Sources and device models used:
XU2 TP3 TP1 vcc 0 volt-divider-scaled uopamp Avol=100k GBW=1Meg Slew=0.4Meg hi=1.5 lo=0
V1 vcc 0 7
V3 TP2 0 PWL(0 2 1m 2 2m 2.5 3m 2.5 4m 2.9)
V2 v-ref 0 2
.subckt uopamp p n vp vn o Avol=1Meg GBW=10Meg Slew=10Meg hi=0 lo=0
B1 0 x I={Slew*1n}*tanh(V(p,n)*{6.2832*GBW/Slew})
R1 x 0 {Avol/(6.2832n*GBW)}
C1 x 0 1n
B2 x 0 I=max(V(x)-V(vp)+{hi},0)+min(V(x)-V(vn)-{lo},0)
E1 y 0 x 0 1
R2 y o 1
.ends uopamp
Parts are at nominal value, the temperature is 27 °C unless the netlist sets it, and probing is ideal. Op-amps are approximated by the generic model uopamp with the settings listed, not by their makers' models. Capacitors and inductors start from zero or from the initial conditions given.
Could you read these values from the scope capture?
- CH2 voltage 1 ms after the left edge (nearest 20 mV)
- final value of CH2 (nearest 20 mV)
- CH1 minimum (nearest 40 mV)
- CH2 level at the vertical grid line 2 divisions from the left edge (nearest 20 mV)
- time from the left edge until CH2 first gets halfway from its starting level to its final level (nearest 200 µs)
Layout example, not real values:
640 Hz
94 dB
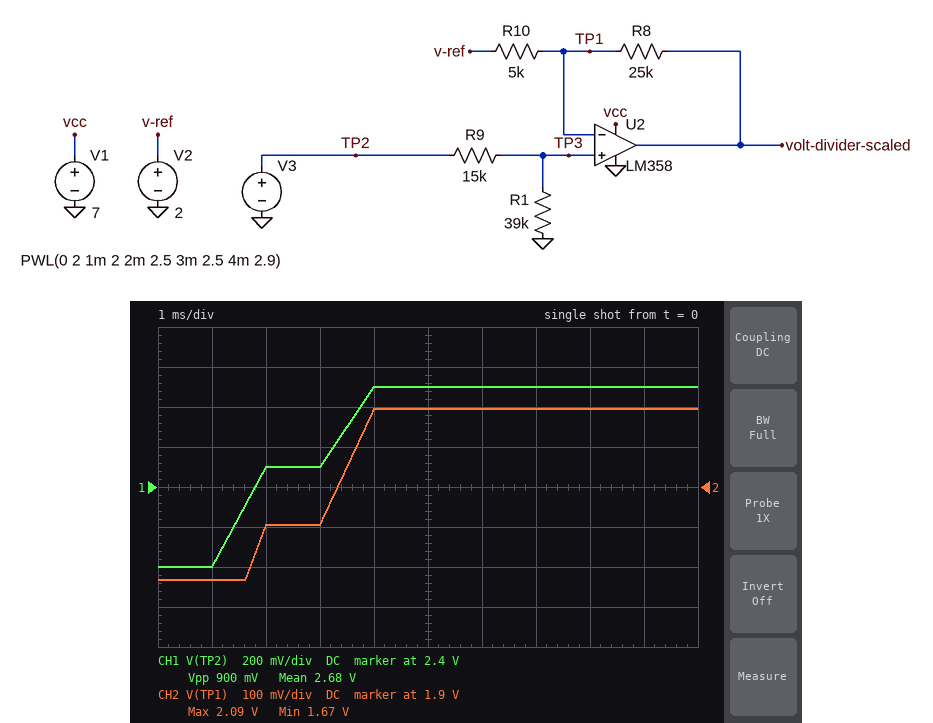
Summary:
1.66 V
2.10 V
2.00 V
1.80 V
3.2 ms
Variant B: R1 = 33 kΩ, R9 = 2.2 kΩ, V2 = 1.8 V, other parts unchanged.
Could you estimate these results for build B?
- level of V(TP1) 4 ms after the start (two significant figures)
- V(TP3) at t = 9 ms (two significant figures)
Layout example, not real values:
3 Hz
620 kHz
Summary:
2.4 V
2.7 V
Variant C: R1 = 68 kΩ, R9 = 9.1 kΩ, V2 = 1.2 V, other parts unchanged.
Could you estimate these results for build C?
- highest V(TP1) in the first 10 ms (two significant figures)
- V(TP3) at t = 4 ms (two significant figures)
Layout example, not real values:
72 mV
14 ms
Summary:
1.9 V
2.6 V
